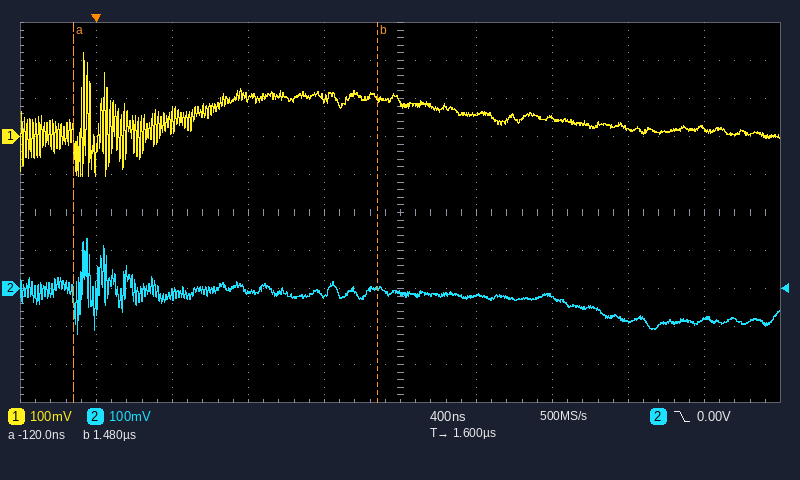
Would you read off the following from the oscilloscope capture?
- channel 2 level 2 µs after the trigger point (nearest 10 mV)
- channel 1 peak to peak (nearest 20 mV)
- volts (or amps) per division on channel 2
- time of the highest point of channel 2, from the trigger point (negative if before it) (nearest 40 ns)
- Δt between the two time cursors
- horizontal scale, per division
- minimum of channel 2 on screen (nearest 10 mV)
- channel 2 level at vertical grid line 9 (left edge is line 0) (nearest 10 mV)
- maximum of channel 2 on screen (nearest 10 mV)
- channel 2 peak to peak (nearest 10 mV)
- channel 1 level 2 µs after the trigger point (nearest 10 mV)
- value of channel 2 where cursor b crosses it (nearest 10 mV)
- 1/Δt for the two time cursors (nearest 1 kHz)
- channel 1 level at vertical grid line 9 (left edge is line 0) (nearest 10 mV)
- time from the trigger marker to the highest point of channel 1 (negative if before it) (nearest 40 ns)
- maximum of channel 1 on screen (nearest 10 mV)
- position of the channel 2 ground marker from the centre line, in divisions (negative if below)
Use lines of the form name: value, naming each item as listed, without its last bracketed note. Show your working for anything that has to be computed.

channel 2 level 2 µs after the trigger point: -20 mV
channel 1 peak to peak: 320 mV
volts (or amps) per division on channel 2: 100 mV
time of the highest point of channel 2, from the trigger point (negative if before it): -40 ns
Δt between the two time cursors: 1.48 µs − (-120 ns) = 1.60 µs
horizontal scale, per division: 400 ns
minimum of channel 2 on screen: -120 mV
channel 2 level at vertical grid line 9 (left edge is line 0): -80 mV
maximum of channel 2 on screen: 130 mV
channel 2 peak to peak: 130 mV − (-120 mV) = 250 mV
channel 1 level 2 µs after the trigger point: 60 mV
value of channel 2 where cursor b crosses it: 0 mV
1/Δt for the two time cursors: 1 / 1.60 µs ≈ 625 kHz
channel 1 level at vertical grid line 9 (left edge is line 0): 20 mV
time from the trigger marker to the highest point of channel 1 (negative if before it): -80 ns
maximum of channel 1 on screen: 220 mV
position of the channel 2 ground marker from the centre line, in divisions: -2.0 div
